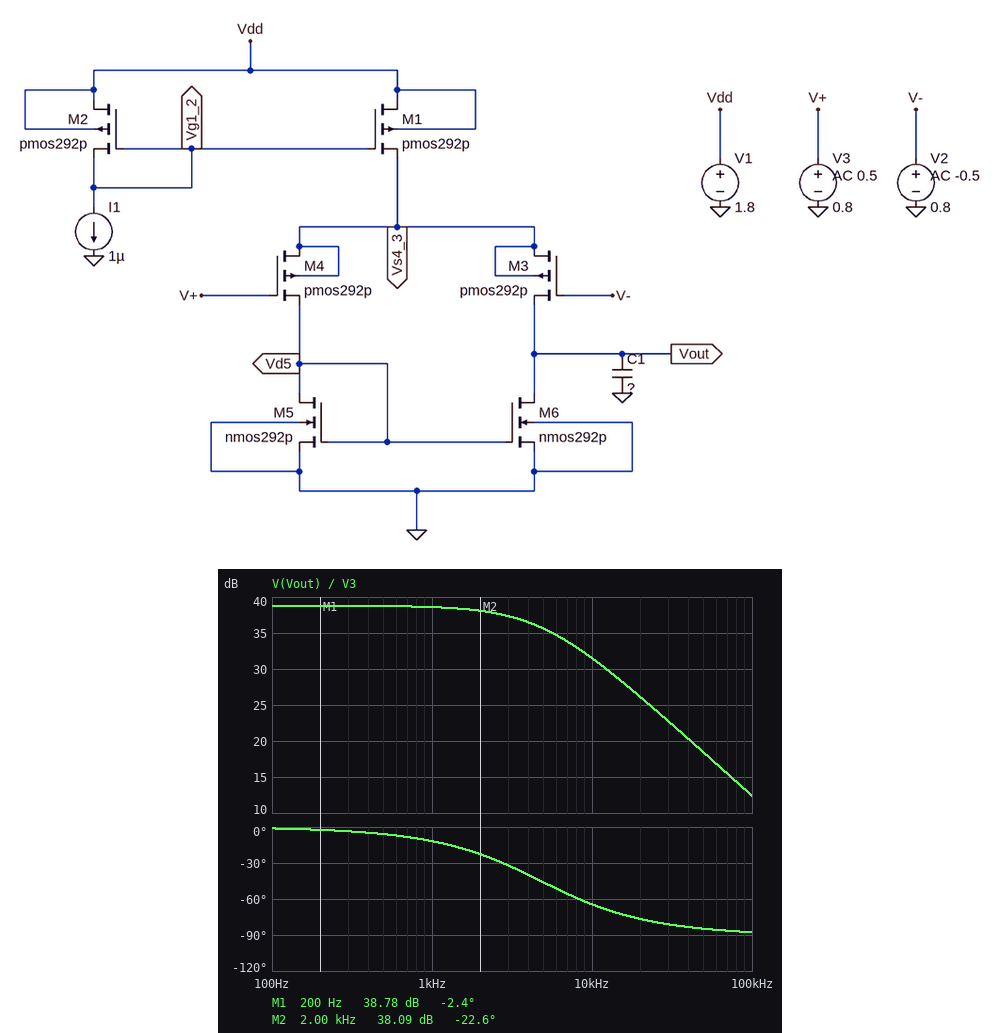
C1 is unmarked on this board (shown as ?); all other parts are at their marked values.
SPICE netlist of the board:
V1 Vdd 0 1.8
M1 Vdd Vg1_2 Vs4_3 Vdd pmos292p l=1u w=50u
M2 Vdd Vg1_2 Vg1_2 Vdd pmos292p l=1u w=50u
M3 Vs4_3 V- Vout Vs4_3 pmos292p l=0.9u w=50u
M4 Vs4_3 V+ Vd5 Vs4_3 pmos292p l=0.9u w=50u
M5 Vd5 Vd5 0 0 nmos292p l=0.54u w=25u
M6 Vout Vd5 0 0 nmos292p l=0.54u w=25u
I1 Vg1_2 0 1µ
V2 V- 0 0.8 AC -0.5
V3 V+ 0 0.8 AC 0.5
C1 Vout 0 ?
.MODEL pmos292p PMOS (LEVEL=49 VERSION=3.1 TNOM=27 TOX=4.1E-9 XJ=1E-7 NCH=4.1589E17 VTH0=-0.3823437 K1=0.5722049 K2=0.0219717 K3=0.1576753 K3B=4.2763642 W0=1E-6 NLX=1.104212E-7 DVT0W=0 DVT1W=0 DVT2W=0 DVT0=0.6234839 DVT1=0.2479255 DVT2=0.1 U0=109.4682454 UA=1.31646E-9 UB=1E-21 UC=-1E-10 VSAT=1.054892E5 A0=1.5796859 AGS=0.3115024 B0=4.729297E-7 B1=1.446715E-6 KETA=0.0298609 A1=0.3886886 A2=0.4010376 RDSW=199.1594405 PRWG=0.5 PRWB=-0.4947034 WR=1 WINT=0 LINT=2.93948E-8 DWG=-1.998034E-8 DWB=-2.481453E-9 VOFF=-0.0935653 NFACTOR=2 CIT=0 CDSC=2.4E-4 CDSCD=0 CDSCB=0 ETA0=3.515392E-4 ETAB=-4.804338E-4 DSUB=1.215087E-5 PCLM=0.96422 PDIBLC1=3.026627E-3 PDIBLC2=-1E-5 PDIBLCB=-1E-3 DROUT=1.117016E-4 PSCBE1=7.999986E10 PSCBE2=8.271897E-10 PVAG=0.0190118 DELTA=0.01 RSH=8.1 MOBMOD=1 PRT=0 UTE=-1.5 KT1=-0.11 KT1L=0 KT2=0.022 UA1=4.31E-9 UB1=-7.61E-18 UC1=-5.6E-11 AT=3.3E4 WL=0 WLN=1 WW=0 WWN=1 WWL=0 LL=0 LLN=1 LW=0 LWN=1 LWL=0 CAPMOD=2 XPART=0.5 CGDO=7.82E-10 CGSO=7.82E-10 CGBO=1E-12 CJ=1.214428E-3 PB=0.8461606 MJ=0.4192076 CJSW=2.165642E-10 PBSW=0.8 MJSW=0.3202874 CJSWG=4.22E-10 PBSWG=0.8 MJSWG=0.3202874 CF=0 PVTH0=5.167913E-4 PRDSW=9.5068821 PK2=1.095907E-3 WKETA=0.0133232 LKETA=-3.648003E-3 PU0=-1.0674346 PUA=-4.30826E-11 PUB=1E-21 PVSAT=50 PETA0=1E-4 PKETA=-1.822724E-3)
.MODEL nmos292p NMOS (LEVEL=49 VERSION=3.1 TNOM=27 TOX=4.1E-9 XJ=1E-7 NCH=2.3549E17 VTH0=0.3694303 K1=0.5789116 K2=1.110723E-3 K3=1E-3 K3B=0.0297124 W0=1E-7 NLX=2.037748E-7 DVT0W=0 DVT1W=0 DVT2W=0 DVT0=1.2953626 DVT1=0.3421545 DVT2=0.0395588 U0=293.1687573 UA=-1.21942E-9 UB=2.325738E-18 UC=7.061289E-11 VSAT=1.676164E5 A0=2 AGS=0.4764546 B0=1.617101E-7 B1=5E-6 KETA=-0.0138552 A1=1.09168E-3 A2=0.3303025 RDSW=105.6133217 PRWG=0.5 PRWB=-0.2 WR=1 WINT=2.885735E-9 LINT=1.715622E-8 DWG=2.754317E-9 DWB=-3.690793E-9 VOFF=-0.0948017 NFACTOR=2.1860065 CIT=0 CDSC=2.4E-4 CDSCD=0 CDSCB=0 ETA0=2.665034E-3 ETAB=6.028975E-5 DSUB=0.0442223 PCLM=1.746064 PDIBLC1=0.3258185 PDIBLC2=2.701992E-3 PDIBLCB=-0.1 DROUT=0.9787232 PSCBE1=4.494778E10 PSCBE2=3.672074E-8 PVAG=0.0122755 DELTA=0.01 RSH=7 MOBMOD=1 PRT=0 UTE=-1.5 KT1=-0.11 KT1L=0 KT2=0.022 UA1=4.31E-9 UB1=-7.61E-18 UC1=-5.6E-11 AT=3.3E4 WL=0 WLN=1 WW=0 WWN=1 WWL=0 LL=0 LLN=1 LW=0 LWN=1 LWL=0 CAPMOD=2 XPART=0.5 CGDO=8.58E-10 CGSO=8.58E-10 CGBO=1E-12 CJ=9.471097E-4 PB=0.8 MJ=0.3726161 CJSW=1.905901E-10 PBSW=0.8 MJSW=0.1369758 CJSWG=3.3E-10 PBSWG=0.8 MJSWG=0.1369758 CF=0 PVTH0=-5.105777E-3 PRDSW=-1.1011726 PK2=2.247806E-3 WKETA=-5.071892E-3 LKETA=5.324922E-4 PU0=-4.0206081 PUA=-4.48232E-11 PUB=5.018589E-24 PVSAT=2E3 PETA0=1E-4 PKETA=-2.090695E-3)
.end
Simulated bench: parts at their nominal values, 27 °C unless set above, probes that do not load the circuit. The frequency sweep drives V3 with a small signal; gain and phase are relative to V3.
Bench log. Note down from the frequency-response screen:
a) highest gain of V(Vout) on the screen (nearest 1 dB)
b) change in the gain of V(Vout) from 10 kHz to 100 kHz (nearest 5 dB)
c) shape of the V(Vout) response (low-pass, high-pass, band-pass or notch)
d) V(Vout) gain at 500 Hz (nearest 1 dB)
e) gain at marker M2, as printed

39 dB
-20 dB
low-pass
39 dB
38.09 dB
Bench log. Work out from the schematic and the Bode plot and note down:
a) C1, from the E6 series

6.8 pF
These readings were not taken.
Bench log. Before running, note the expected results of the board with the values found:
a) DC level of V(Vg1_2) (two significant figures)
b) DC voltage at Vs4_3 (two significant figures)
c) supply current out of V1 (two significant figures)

1.4 V
1.1 V
2.0 µA
